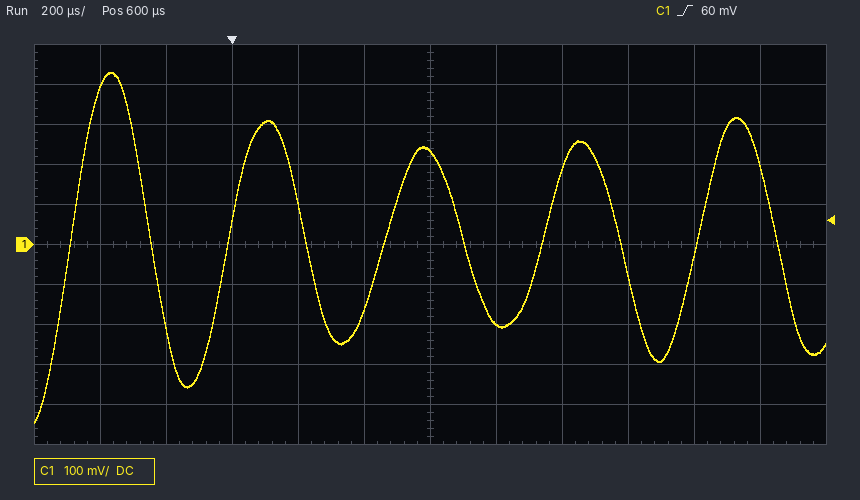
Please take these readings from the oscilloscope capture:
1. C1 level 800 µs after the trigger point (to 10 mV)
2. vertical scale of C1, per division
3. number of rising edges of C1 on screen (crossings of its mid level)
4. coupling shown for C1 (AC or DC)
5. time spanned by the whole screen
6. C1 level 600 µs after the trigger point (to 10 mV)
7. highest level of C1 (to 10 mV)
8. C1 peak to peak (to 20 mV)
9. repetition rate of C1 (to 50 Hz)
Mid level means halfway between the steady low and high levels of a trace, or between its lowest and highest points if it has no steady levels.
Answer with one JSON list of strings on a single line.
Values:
["-200 mV", "100 mV", "5", "DC", "2.4 ms", "230 mV", "430 mV", "880 mV", "2.10 kHz"]
